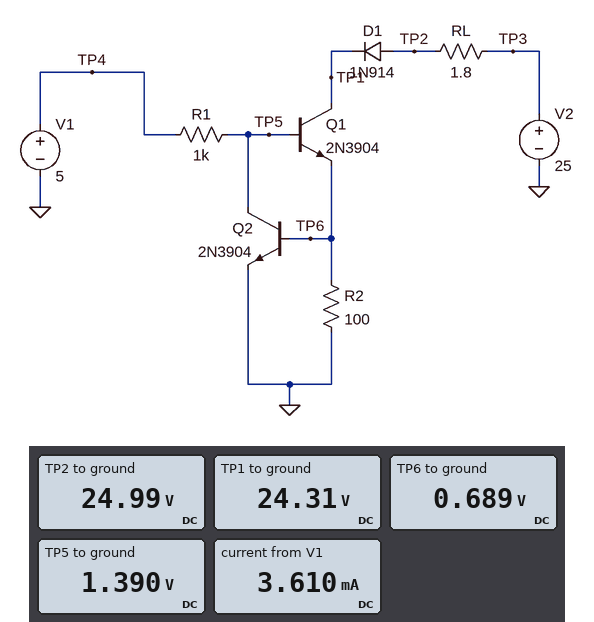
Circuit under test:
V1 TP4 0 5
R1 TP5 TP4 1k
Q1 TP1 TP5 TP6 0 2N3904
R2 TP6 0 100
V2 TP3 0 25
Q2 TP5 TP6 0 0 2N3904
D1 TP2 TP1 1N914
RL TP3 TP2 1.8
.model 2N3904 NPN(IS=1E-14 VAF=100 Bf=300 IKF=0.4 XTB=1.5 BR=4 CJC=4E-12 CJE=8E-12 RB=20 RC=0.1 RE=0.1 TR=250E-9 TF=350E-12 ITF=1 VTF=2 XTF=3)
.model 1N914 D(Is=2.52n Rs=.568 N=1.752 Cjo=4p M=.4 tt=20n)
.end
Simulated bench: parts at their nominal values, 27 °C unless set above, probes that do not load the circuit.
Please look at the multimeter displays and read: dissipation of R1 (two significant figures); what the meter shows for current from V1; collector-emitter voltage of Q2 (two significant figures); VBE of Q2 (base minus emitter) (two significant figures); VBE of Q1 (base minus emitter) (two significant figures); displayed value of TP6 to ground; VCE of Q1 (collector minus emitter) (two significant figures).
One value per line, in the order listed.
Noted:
13 mW
3.610 mA
1.4 V
690 mV
700 mV
0.689 V
24 V
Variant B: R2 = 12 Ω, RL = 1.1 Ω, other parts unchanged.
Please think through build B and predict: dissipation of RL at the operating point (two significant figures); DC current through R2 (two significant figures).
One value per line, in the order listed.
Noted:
3.6 mW
57 mA
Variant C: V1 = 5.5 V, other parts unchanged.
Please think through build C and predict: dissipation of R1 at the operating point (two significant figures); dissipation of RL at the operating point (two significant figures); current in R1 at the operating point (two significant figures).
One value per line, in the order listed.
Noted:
17 mW
86 µW
4.1 mA
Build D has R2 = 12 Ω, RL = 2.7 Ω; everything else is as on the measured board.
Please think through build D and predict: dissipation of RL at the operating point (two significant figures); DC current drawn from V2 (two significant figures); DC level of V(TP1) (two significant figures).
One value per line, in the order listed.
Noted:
8.8 mW
57 mA
24 V
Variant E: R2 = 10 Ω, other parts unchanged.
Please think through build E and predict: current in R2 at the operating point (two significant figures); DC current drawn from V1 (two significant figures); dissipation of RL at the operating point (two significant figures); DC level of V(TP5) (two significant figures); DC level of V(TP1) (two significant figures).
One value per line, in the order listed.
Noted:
69 mA
3.5 mA
8.4 mW
1.5 V
24 V
